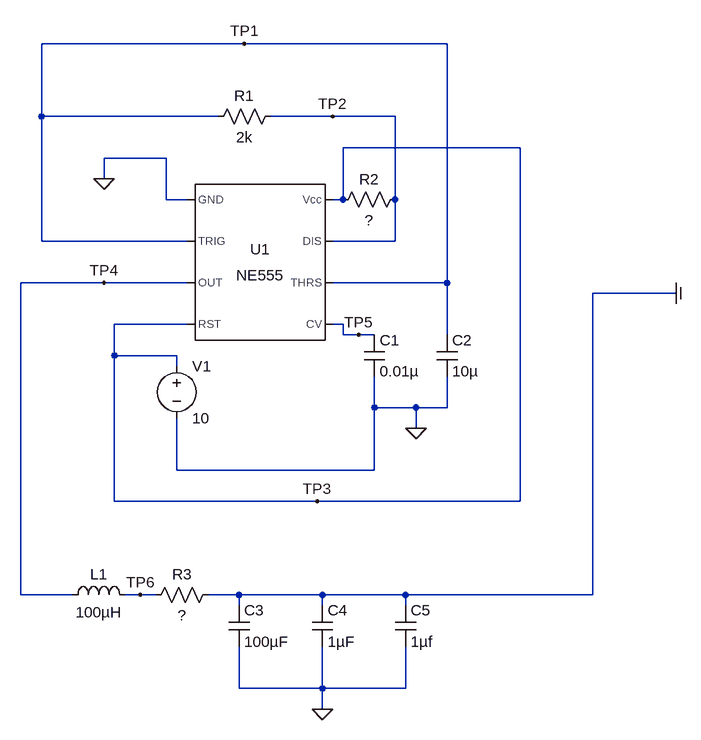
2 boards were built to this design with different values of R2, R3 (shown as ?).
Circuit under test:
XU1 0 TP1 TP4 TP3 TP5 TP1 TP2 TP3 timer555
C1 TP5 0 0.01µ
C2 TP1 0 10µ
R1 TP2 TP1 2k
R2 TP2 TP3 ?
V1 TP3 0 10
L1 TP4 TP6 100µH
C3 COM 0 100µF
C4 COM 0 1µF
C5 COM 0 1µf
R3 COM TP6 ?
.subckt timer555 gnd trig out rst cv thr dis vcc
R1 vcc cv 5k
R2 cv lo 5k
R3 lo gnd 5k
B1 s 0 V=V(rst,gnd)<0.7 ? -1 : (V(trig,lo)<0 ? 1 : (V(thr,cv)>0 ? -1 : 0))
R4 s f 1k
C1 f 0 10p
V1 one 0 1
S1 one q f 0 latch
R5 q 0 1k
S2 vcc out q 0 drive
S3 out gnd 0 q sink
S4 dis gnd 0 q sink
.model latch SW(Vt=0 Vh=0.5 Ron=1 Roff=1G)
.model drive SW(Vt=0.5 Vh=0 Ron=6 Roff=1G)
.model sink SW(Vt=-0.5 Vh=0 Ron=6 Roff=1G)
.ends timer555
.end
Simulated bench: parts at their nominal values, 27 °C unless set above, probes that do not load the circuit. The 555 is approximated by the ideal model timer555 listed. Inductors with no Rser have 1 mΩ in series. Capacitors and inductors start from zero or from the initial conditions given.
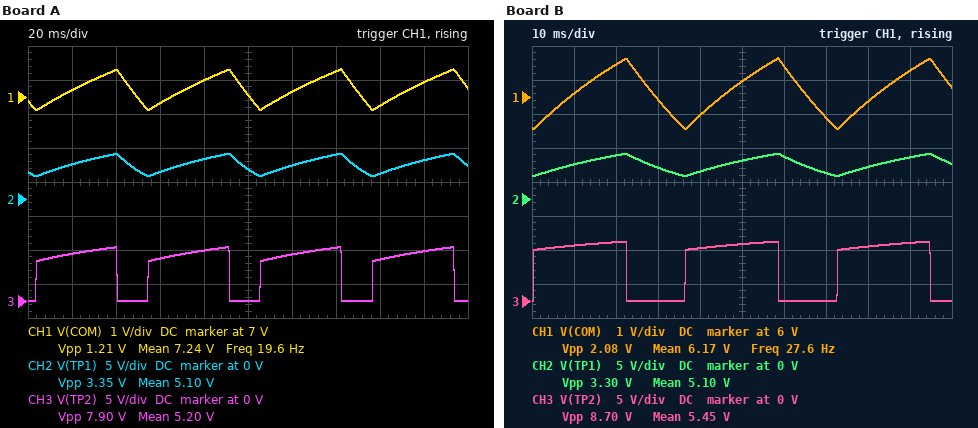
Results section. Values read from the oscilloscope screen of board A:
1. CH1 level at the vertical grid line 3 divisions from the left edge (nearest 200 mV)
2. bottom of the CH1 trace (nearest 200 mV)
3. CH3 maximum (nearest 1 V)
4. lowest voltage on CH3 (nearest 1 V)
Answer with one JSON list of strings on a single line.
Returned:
["6.8 V", "6.6 V", "8 V", "0 V"]
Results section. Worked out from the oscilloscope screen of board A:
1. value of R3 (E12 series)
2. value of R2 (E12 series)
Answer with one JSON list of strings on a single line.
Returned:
["820 Ω", "3.3 kΩ"]
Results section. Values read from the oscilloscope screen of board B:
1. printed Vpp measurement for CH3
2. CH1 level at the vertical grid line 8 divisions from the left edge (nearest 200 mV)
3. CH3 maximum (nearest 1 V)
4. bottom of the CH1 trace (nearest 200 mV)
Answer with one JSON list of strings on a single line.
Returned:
["8.70 V", "5.8 V", "9 V", "5.0 V"]
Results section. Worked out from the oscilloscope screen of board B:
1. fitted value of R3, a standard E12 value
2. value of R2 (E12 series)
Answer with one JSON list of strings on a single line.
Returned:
["390 Ω", "1.2 kΩ"]
